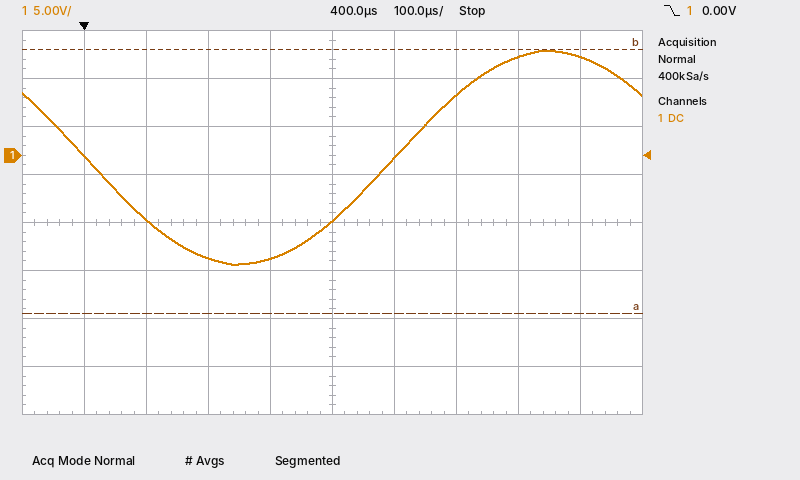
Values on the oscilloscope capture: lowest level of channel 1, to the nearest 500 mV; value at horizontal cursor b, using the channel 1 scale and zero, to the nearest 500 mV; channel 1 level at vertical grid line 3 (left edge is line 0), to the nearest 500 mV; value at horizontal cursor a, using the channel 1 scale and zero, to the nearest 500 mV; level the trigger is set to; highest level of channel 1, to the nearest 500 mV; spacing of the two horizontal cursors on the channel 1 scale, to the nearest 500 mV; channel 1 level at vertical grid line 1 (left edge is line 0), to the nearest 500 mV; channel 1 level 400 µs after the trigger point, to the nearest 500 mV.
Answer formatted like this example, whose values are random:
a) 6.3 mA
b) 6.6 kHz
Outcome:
a) -11.5 V
b) 11.0 V
c) -10.5 V
d) -16.5 V
e) 0.00 V
f) 11.0 V
g) 27.5 V
h) 0.0 V
i) -7.0 V
